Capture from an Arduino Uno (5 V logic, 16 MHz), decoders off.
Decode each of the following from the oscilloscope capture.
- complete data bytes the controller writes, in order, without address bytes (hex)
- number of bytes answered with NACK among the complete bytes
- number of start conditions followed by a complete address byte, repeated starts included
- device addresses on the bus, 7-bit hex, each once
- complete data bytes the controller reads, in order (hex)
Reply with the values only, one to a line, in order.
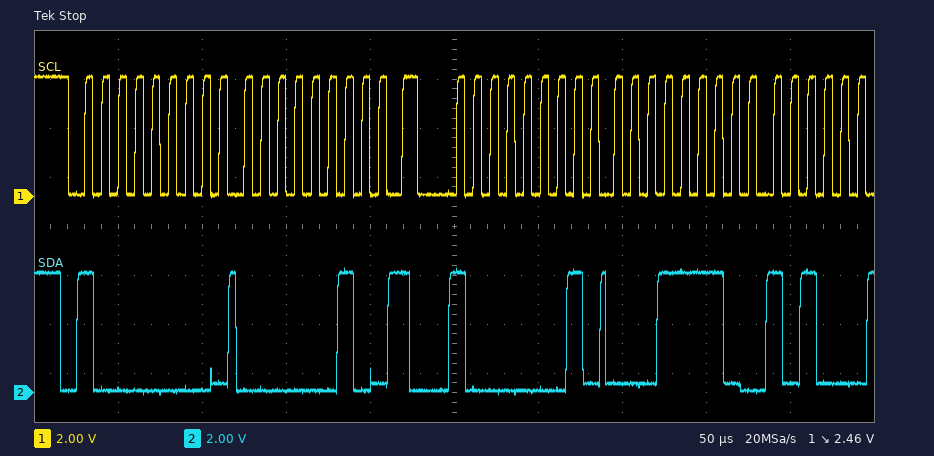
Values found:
02
0
2
0x40
1E
